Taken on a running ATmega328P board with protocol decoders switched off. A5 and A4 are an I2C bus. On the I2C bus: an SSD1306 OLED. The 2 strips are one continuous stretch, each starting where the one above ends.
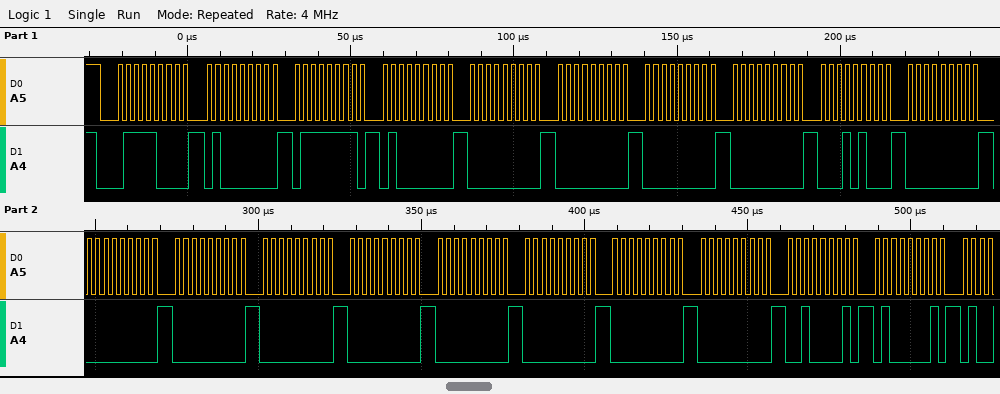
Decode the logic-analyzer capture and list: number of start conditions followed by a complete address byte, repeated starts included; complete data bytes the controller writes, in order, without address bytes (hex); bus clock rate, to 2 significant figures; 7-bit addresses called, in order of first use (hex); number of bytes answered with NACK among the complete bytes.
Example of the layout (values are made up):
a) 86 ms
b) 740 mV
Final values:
a) 1
b) 40 7F 40 00 00 00 00 14 00 00 00 00 00 00 00 00 00 21 41
c) 400 kHz
d) 0x3C
e) 0
